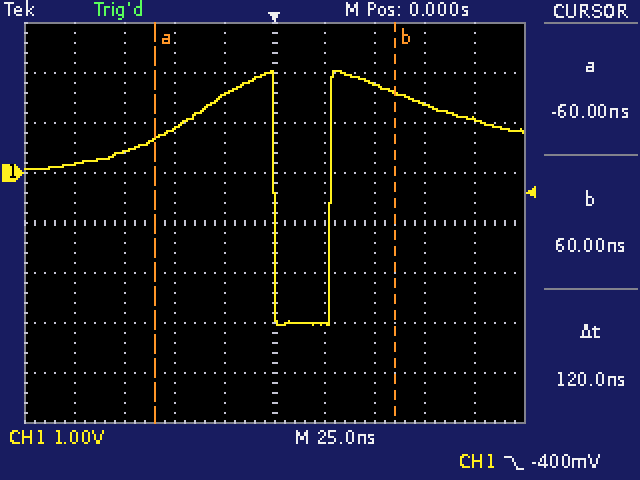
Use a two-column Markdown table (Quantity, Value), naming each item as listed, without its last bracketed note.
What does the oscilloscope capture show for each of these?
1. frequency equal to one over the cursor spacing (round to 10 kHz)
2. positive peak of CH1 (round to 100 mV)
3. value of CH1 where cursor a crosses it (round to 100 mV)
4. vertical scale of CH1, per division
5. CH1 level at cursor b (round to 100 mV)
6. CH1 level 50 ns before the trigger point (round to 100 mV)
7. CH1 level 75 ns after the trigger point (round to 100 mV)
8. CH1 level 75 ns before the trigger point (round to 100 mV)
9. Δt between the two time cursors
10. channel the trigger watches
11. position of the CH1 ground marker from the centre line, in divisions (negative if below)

| Quantity | Value |
|---|---|
| frequency equal to one over the cursor spacing | 8.33 MHz |
| positive peak of CH1 | 2.0 V |
| value of CH1 where cursor a crosses it | 700 mV |
| vertical scale of CH1, per division | 1 V |
| CH1 level at cursor b | 1.6 V |
| CH1 level 50 ns before the trigger point | 900 mV |
| CH1 level 75 ns after the trigger point | 1.4 V |
| CH1 level 75 ns before the trigger point | 400 mV |
| Δt between the two time cursors | 120 ns |
| channel the trigger watches | CH1 |
| position of the CH1 ground marker from the centre line, in divisions | +1.0 div |
